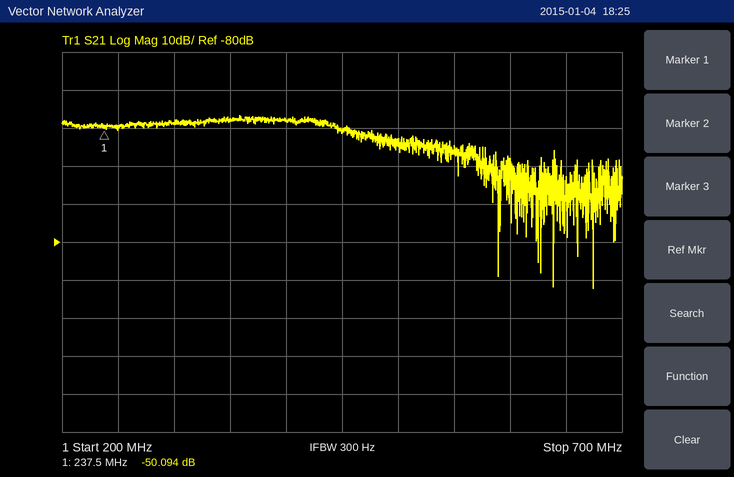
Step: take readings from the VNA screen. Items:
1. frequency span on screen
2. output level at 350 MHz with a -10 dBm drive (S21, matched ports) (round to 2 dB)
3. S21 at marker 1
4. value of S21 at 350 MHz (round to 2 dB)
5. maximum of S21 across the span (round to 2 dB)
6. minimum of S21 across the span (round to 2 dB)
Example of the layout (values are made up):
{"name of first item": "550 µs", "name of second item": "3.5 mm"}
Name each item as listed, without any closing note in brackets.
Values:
{"frequency span on screen": "500 MHz", "output level at 350 MHz with a -10 dBm drive (S21, matched ports)": "-58 dBm", "S21 at marker 1": "-50.094 dB", "value of S21 at 350 MHz": "-48 dB", "maximum of S21 across the span": "-46 dB", "minimum of S21 across the span": "-92 dB"}
